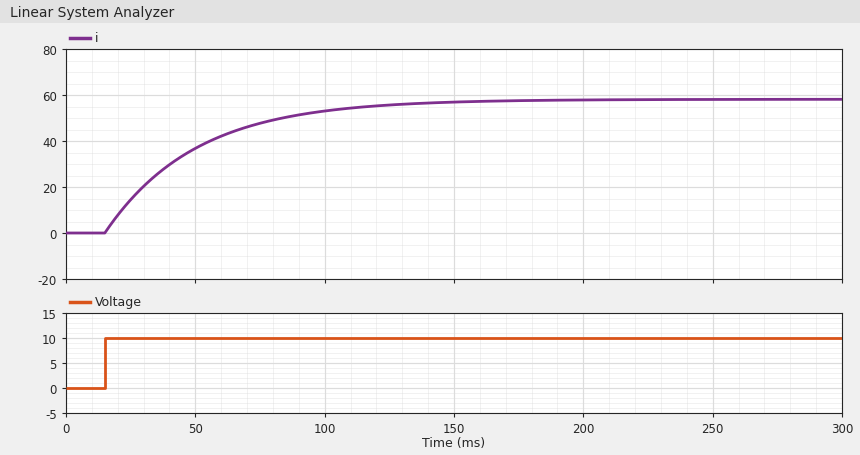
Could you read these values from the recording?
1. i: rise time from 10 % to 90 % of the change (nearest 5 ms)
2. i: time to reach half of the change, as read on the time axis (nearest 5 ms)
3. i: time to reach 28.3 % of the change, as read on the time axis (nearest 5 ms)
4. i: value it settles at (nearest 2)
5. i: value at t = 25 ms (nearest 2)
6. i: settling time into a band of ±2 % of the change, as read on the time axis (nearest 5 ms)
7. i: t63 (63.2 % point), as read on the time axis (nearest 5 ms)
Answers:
75 ms
40 ms
25 ms
58
14
150 ms
50 ms
